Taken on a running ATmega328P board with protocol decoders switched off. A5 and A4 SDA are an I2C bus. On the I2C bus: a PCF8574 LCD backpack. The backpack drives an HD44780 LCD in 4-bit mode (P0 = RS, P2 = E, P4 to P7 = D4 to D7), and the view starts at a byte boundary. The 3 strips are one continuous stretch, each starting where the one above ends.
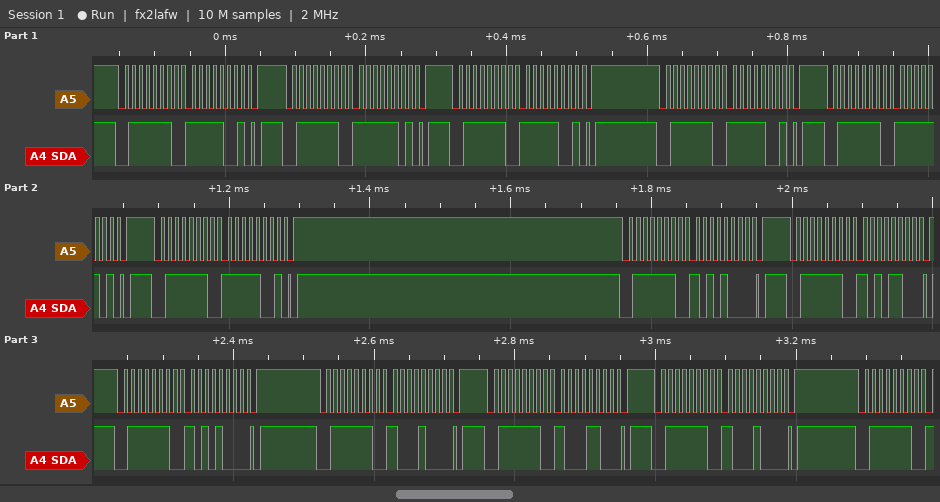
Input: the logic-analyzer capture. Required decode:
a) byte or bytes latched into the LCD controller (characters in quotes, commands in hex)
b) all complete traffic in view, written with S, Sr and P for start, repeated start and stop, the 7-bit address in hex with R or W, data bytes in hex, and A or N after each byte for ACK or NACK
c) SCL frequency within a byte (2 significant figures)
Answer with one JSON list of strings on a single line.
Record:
["data 0xFF 0xA8", "S 3FW A F9 A P S 3FW A FD A P S 3FW A F9 A P S 3FW A F9 A P S 3FW A FD A P S 3FW A F9 A P S 3FW A A8 A P S 3FW A AC A P S 3FW A A8 A P S 3FW A 88 A P S 3FW A 8C A P S 3FW A 88 A P S 3FW A", "100 kHz"]
